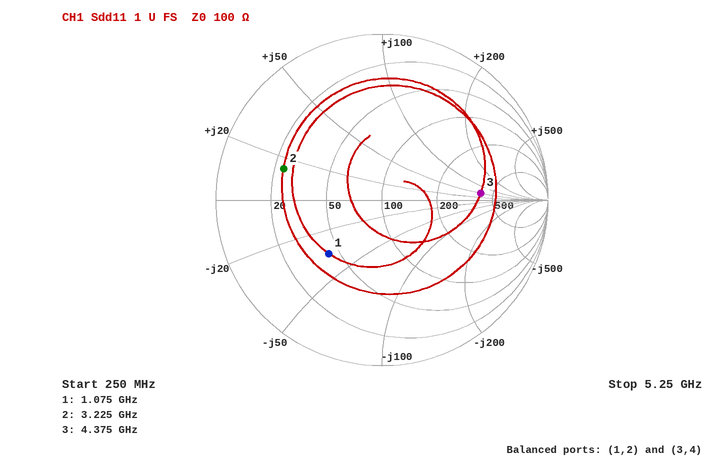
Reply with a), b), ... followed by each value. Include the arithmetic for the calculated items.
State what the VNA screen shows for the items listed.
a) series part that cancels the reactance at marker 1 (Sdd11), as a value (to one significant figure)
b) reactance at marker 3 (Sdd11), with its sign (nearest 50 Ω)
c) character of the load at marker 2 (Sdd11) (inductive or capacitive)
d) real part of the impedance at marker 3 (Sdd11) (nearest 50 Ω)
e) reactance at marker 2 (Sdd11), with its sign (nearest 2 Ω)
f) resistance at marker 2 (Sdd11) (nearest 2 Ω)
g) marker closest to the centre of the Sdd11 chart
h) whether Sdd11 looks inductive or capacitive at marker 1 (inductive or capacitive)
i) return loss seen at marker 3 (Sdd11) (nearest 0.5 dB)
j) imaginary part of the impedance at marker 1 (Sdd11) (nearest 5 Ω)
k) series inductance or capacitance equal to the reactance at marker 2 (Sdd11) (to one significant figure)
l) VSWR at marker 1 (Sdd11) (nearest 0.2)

a) L = 35 Ω/(2π × 1.075 GHz) ≈ 5 nH
b) +50 Ω
c) inductive
d) 400 Ω
e) +14 Ω
f) 24 Ω
g) marker 1
h) capacitive
i) 4.5 dB
j) -35 Ω
k) L = 14 Ω/(2π × 3.225 GHz) ≈ 691 pH, so 700 pH to one significant figure
l) 2.6
